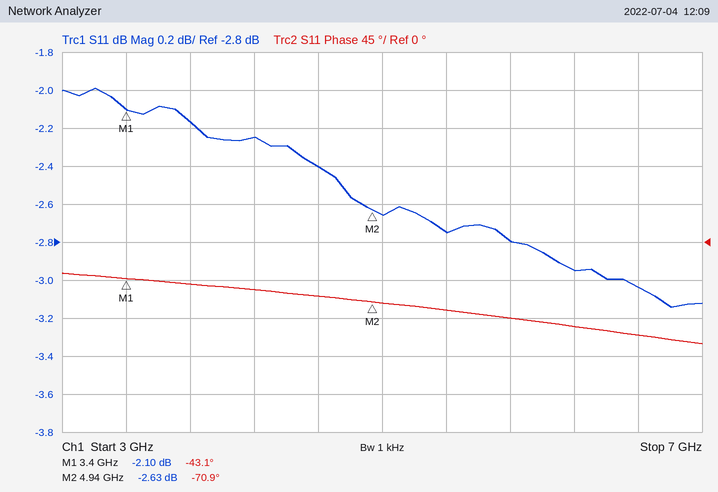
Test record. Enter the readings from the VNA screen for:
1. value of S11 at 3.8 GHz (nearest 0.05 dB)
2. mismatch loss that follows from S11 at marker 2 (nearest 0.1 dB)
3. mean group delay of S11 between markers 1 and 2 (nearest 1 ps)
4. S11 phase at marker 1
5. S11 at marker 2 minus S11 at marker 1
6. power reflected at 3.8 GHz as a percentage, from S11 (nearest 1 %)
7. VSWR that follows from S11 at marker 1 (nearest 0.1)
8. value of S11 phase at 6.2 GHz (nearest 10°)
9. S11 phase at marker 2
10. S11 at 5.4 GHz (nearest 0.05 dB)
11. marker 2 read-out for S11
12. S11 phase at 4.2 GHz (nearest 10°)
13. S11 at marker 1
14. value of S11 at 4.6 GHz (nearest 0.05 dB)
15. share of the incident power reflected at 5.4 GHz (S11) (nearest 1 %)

-2.15 dB
3.4 dB
50 ps
-43.1°
-0.53 dB
61 %
8.3
-100°
-70.9°
-2.75 dB
-2.63 dB
-60°
-2.10 dB
-2.40 dB
53 %
